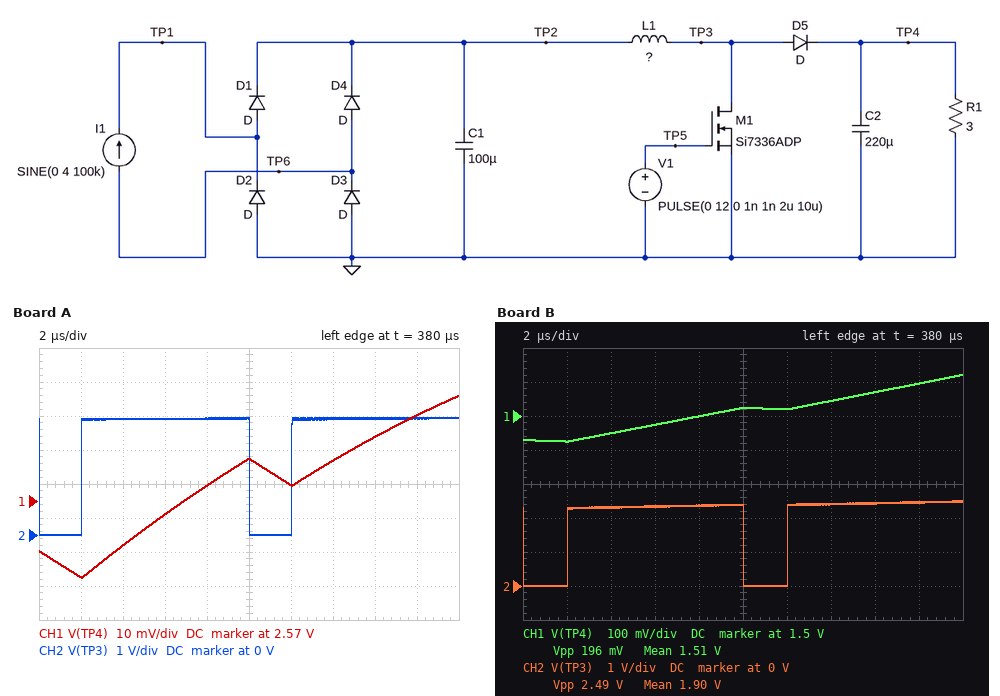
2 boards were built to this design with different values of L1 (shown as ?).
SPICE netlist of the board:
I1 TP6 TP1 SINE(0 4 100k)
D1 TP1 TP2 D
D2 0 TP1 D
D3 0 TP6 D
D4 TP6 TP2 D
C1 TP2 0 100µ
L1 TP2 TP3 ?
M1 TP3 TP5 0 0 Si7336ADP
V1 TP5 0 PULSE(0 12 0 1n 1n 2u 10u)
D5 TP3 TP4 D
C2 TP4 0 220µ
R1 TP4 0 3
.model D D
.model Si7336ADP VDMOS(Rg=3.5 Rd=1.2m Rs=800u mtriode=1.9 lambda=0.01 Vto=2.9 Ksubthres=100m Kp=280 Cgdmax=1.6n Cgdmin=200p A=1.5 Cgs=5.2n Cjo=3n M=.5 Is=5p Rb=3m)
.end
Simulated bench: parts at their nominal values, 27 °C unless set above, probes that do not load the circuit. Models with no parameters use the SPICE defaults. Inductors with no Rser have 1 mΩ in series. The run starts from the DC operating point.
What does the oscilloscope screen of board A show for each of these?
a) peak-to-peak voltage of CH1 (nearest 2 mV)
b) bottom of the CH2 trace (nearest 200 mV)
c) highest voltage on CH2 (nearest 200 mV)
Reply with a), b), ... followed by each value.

a) 54 mV
b) 0 V
c) 3.4 V
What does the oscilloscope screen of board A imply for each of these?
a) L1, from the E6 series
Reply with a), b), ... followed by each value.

a) 68 µH
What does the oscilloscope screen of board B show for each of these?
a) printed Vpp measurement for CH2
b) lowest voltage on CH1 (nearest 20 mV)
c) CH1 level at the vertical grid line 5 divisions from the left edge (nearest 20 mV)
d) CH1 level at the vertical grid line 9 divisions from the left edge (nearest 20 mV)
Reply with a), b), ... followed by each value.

a) 2.49 V
b) 1.42 V
c) 1.52 V
d) 1.60 V
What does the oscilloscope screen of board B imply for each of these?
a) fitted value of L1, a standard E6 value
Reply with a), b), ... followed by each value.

a) 330 µH
